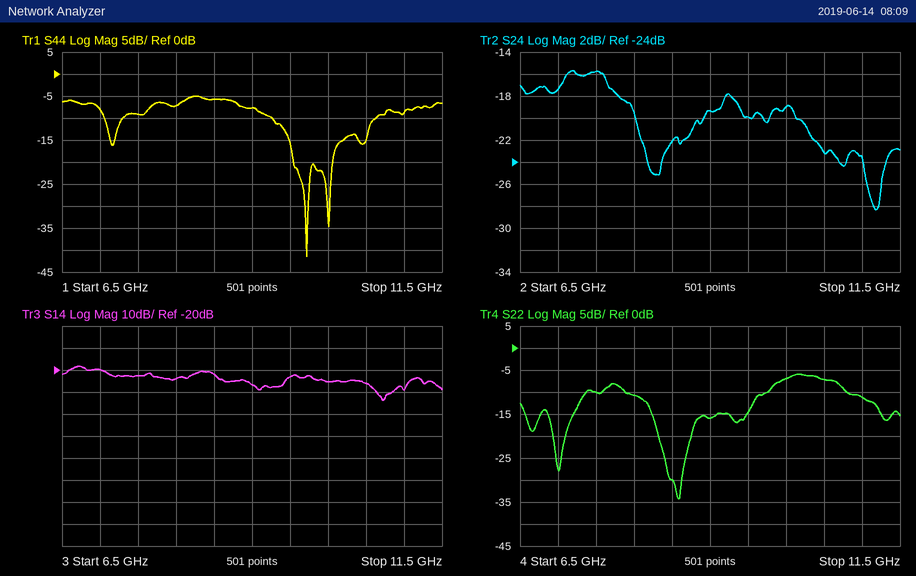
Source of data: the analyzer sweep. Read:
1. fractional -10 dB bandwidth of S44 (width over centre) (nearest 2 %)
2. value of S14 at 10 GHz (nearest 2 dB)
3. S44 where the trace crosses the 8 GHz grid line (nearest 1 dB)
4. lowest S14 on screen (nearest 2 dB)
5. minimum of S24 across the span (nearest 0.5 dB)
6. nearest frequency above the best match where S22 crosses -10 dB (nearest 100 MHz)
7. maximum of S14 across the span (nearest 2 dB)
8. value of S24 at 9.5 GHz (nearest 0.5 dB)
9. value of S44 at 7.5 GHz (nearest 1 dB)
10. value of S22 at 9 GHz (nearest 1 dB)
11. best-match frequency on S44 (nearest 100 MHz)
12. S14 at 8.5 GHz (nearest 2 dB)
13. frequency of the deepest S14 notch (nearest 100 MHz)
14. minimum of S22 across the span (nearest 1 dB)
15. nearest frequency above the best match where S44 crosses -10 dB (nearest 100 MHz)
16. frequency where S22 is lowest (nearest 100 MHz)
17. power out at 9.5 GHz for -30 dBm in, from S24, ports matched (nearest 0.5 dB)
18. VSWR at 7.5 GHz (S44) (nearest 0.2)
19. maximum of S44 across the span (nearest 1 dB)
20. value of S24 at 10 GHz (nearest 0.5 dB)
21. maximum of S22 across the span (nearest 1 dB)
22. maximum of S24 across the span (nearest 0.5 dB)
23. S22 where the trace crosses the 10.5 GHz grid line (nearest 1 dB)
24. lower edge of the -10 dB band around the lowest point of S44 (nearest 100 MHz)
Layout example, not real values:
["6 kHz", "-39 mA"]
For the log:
["14 %", "-26 dB", "-7 dB", "-34 dB", "-28.5 dB", "9.8 GHz", "-18 dB", "-20.0 dB", "-9 dB", "-16 dB", "9.7 GHz", "-22 dB", "10.7 GHz", "-34 dB", "10.6 GHz", "8.6 GHz", "-50.0 dBm", "2.0", "-5 dB", "-19.0 dB", "-6 dB", "-15.5 dB", "-7 dB", "9.3 GHz"]
